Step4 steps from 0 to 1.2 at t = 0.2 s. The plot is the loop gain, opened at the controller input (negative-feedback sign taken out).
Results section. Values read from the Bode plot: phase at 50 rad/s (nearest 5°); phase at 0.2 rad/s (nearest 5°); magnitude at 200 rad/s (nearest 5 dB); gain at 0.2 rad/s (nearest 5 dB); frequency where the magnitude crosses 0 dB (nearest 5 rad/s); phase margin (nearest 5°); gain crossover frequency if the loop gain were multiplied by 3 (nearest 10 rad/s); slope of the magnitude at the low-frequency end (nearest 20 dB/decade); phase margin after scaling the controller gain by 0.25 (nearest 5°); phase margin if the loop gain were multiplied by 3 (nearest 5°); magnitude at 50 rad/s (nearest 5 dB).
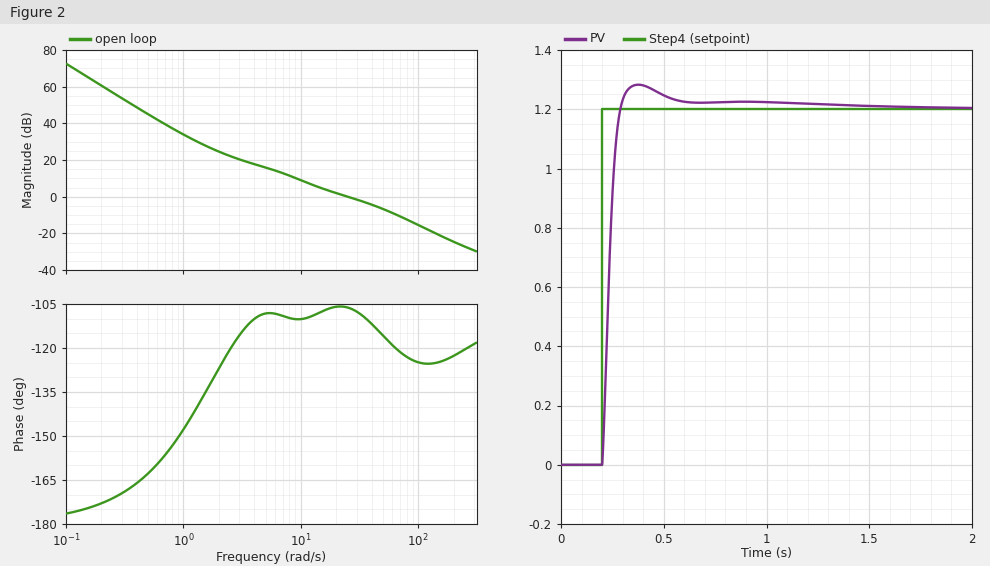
-115°
-175°
-25 dB
60 dB
25 rad/s
75°
60 rad/s
-40 dB/decade
70°
60°
-5 dB
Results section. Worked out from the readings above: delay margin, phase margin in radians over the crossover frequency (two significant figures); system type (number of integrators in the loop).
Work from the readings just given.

0.052 s
2
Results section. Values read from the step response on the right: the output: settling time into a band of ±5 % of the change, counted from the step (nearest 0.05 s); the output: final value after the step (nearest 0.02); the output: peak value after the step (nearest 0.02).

0.25 s
1.20
1.28
